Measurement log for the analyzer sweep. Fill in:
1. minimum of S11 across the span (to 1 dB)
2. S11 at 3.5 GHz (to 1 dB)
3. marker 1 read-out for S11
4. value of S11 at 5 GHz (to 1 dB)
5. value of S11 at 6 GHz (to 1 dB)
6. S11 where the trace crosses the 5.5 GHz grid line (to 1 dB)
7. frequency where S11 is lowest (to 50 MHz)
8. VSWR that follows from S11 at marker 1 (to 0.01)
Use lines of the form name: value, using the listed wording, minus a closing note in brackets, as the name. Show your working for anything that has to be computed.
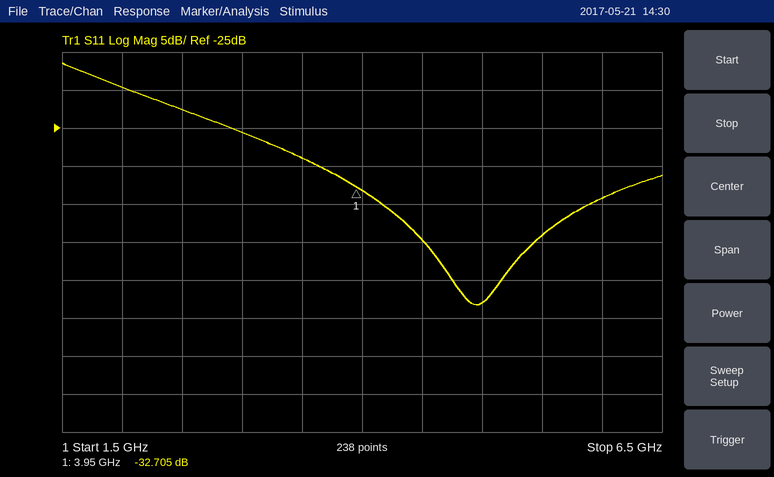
minimum of S11 across the span: -48 dB
S11 at 3.5 GHz: -29 dB
marker 1 read-out for S11: -32.705 dB
value of S11 at 5 GHz: -48 dB
value of S11 at 6 GHz: -34 dB
S11 where the trace crosses the 5.5 GHz grid line: -39 dB
frequency where S11 is lowest: 4.95 GHz
VSWR that follows from S11 at marker 1: (1 + 0.0232)/(1 − 0.0232) ≈ 1.05
